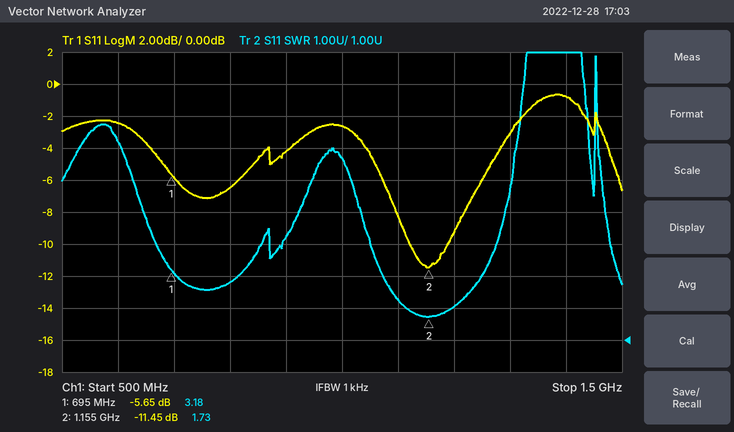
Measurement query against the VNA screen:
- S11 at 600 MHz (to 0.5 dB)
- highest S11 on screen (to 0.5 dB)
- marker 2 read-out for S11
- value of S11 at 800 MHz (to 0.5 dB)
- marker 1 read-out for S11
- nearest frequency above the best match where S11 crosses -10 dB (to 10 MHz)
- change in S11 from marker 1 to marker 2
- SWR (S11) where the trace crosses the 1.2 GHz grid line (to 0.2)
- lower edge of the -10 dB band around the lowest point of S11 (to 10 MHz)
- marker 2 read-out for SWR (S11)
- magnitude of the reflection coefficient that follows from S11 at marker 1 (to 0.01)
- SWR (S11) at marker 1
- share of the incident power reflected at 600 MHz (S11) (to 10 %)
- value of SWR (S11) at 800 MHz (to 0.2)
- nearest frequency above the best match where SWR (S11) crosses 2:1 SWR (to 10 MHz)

-2.5 dB
-0.5 dB
-11.45 dB
-6.5 dB
-5.65 dB
1.19 GHz
-5.80 dB
2.0
1.12 GHz
1.73
0.52
3.18
60 %
2.8
1.20 GHz
